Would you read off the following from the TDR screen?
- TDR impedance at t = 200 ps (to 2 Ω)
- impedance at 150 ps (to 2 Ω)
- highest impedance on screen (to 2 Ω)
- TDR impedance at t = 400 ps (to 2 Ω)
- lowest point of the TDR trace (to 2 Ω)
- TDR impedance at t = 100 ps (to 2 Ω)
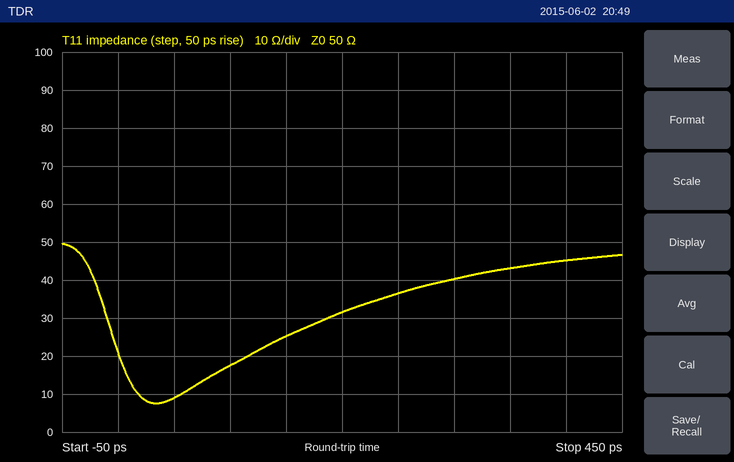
32 Ω
26 Ω
50 Ω
46 Ω
8 Ω
18 Ω
